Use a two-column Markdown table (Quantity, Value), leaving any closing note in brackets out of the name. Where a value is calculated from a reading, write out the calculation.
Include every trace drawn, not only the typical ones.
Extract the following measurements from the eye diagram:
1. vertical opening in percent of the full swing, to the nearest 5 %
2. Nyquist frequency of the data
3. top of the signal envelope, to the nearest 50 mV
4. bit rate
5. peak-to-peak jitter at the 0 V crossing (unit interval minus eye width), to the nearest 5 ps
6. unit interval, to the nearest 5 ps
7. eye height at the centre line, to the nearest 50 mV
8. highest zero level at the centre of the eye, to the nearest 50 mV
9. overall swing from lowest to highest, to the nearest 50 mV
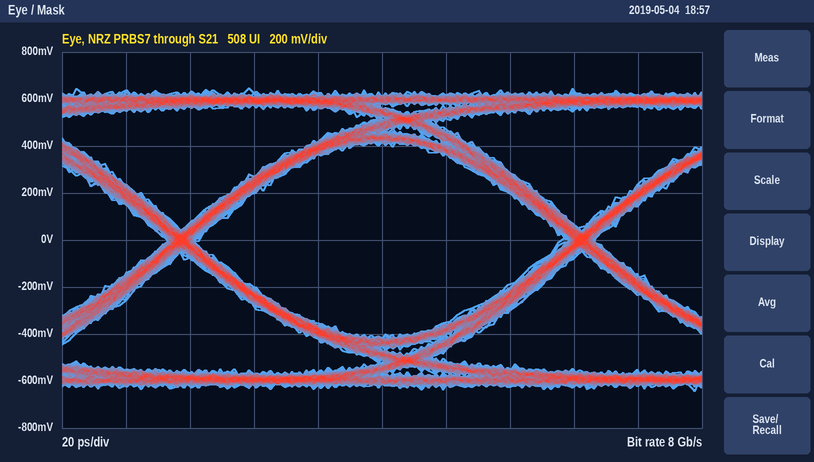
| Quantity | Value |
|---|---|
| vertical opening in percent of the full swing, to the nearest 5 % | 850 mV / 1.30 V ≈ 65 % |
| Nyquist frequency of the data | 4 GHz |
| top of the signal envelope, to the nearest 50 mV | 650 mV |
| bit rate | 8 Gb/s |
| peak-to-peak jitter at the 0 V crossing (unit interval minus eye width), to the nearest 5 ps | 10 ps |
| unit interval, to the nearest 5 ps | 125 ps |
| eye height at the centre line, to the nearest 50 mV | 850 mV |
| highest zero level at the centre of the eye, to the nearest 50 mV | -400 mV |
| overall swing from lowest to highest, to the nearest 50 mV | 1.30 V |
